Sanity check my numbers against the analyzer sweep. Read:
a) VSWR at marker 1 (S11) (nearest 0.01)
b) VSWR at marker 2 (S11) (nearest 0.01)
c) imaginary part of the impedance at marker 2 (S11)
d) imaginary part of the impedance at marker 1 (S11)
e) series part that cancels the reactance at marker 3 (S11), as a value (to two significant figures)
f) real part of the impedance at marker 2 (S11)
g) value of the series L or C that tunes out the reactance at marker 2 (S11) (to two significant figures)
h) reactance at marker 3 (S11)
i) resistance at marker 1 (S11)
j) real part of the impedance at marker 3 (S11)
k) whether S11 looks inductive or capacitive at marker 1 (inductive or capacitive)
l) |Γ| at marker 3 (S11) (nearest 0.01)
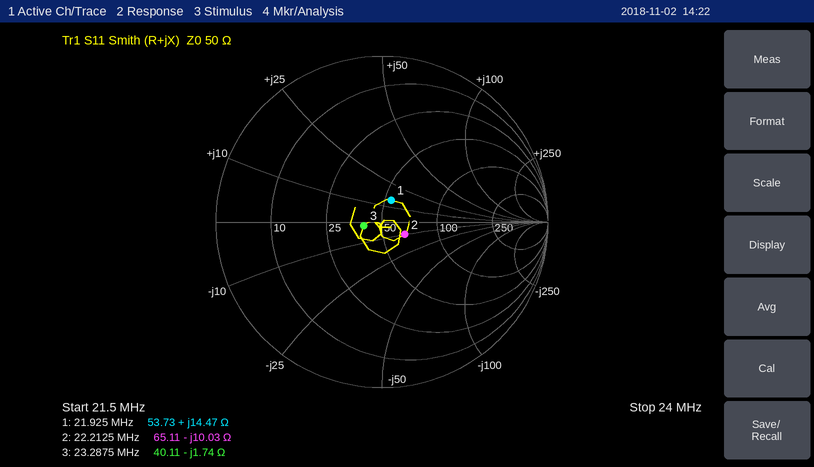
1.33
1.37
-10.03 Ω
+14.47 Ω
12 nH
65.11 Ω
72 nH
-1.74 Ω
53.73 Ω
40.11 Ω
inductive
0.11
